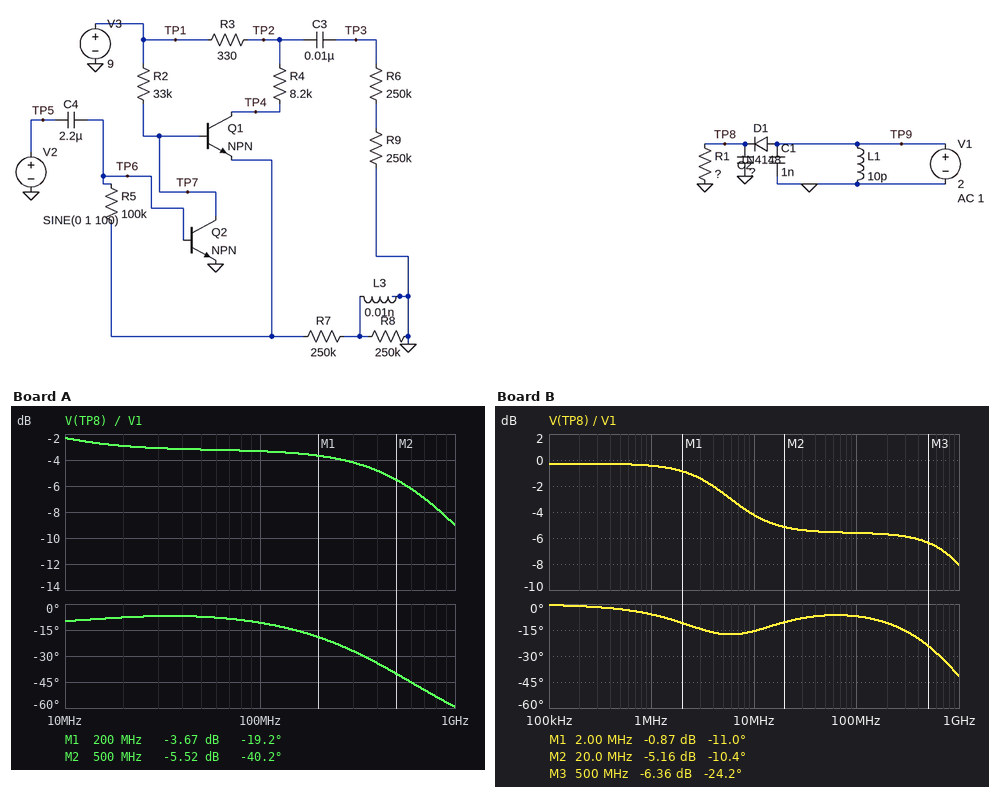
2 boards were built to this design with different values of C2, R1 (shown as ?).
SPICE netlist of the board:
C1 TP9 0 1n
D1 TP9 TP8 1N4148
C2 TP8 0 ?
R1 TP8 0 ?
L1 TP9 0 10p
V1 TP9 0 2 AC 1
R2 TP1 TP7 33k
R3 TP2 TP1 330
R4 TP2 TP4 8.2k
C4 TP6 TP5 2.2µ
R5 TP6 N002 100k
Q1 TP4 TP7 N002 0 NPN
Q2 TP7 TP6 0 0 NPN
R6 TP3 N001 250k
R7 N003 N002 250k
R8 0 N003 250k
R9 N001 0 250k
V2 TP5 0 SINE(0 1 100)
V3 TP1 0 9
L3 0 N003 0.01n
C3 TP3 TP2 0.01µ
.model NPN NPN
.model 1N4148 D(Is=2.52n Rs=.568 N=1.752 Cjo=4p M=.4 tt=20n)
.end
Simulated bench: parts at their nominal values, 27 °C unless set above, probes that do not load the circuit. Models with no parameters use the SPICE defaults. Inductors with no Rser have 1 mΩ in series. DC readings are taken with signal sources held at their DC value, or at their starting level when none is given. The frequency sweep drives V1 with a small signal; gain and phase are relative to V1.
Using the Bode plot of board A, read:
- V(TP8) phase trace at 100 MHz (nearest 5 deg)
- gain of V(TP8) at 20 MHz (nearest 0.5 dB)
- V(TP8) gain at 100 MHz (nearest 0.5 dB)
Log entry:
-10 deg
-3.0 dB
-3.5 dB
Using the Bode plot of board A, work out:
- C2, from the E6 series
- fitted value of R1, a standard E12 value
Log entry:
680 pF
390 Ω
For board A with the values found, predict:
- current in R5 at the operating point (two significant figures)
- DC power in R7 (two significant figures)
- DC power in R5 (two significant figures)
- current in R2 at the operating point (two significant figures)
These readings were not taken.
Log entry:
2.2 µA
3.7 µW
500 nW
220 µA
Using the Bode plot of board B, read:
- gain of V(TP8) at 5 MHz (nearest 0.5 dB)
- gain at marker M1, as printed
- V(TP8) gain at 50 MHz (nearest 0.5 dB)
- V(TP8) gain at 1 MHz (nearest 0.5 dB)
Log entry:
-2.5 dB
-0.87 dB
-5.5 dB
-0.5 dB
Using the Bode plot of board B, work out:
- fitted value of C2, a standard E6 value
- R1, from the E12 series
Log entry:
470 pF
1.2 kΩ
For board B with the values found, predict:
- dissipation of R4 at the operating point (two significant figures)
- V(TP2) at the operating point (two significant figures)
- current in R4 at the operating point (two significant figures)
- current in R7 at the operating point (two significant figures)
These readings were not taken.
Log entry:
300 nW
9.0 V
6.0 µA
3.8 µA
